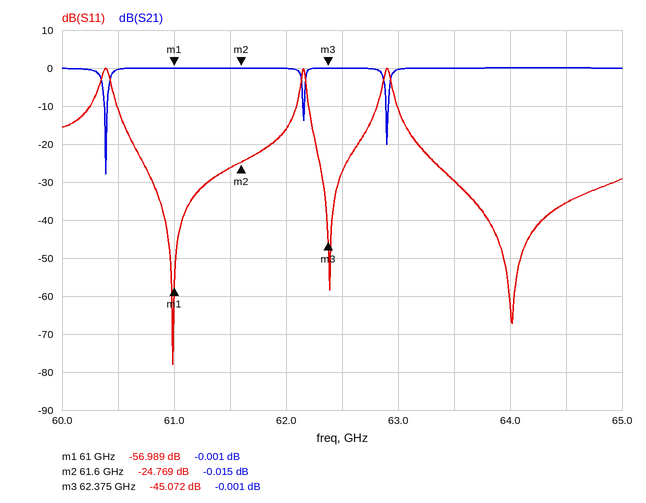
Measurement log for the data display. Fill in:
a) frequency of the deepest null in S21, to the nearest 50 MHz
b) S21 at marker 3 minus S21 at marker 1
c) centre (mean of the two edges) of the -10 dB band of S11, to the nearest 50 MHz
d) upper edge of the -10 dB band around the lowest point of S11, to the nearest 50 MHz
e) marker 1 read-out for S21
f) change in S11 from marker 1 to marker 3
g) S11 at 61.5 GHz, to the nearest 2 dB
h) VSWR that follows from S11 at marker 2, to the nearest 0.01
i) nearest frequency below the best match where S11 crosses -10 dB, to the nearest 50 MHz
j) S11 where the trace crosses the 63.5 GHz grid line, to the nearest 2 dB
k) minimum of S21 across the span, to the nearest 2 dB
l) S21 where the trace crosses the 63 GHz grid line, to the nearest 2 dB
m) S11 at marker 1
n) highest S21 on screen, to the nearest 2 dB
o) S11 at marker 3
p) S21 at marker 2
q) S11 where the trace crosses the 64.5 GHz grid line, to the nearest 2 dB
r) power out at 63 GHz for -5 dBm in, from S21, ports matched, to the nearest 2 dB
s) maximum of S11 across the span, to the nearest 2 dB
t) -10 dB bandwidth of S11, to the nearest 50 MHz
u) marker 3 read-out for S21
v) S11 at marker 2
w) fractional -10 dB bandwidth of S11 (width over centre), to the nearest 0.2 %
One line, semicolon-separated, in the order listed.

60.40 GHz; 0.000 dB; 61.30 GHz; 62.10 GHz; -0.001 dB; 11.917 dB; -26 dB; 1.12; 60.50 GHz; -30 dB; -28 dB; 0 dB; -56.989 dB; 0 dB; -45.072 dB; -0.015 dB; -36 dB; -6 dBm; 0 dB; 1.60 GHz; -0.001 dB; -24.769 dB; 2.6 %
